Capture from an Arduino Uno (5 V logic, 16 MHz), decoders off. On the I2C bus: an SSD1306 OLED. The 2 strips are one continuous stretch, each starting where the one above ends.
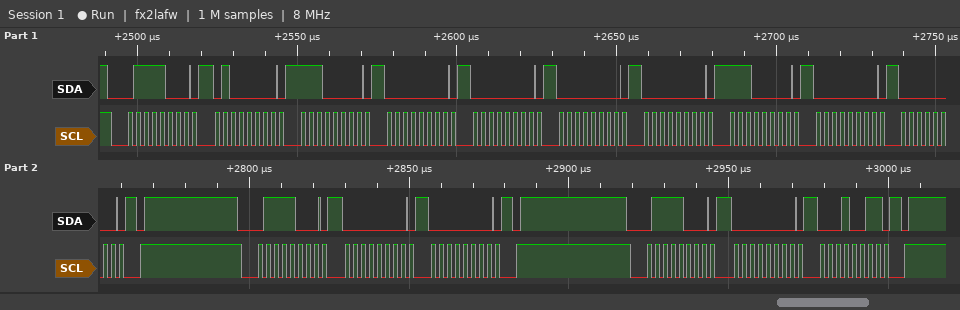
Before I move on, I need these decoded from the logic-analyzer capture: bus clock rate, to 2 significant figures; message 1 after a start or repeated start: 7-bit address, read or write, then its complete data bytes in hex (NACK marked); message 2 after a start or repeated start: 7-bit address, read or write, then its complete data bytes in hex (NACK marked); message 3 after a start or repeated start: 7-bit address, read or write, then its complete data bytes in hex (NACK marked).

400 kHz
0x3C write: 40 E0 00 00 00 00 E0 00 00
0x3C write: 00 00
0x3C write: 00 13
